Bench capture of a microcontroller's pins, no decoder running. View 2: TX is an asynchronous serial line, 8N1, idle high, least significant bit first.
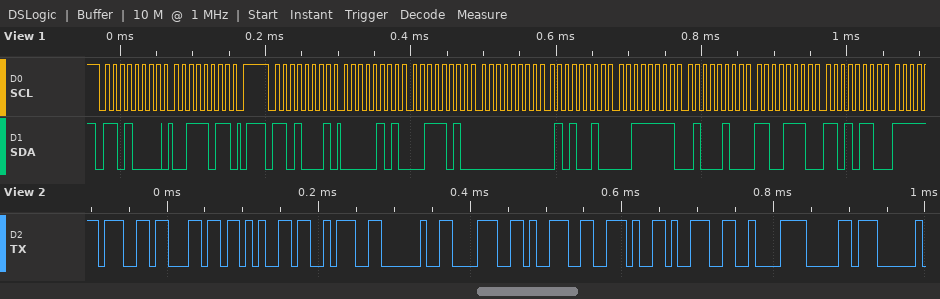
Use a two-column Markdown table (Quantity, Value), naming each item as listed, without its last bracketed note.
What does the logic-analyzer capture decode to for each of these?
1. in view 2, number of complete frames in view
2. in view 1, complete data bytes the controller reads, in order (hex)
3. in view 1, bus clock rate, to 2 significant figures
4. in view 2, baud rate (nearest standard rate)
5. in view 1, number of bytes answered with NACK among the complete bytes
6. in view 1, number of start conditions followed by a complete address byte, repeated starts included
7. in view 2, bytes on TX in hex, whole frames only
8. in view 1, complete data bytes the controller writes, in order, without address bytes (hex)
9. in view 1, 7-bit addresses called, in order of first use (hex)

| Quantity | Value |
|---|---|
| in view 2, number of complete frames in view | 11 |
| in view 1, complete data bytes the controller reads, in order | 05 3A 00 52 3F 44 CE D6 |
| in view 1, bus clock rate, to 2 significant figures | 100 kHz |
| in view 2, baud rate | 115200 baud |
| in view 1, number of bytes answered with NACK among the complete bytes | 0 |
| in view 1, number of start conditions followed by a complete address byte, repeated starts included | 2 |
| in view 2, bytes on TX in hex, whole frames only | 67 6C 65 3A 20 38 39 2E 39 C2 B0 |
| in view 1, complete data bytes the controller writes, in order, without address bytes | 3B |
| in view 1, 7-bit addresses called, in order of first use | 0x68 |
